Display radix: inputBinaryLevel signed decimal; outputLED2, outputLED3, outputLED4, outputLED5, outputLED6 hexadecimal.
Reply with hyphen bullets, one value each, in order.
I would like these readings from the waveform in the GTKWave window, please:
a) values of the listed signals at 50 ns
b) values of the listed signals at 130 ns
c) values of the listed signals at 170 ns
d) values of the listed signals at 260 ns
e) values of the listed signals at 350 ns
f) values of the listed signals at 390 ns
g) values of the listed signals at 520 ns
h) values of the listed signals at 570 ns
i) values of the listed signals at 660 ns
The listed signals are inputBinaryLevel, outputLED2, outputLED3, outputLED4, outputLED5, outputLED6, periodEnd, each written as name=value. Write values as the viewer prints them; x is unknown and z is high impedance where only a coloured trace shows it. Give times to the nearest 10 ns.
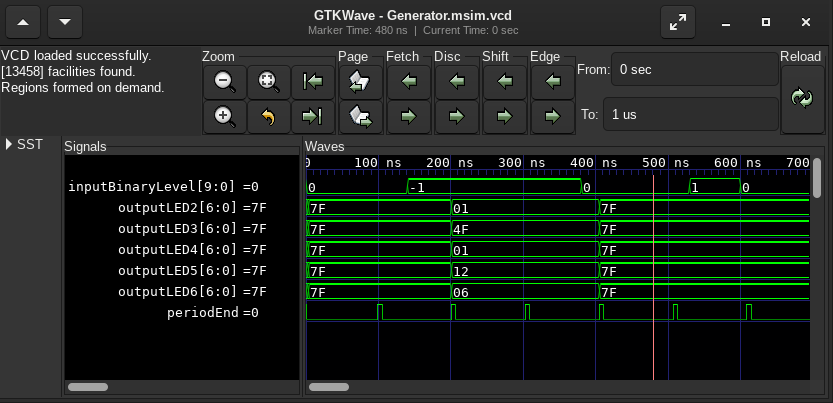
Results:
- inputBinaryLevel=0, outputLED2=7F, outputLED3=7F, outputLED4=7F, outputLED5=7F, outputLED6=7F, periodEnd=0
- inputBinaryLevel=0, outputLED2=7F, outputLED3=7F, outputLED4=7F, outputLED5=7F, outputLED6=7F, periodEnd=0
- inputBinaryLevel=-1, outputLED2=7F, outputLED3=7F, outputLED4=7F, outputLED5=7F, outputLED6=7F, periodEnd=0
- inputBinaryLevel=-1, outputLED2=01, outputLED3=4F, outputLED4=01, outputLED5=12, outputLED6=06, periodEnd=0
- inputBinaryLevel=-1, outputLED2=01, outputLED3=4F, outputLED4=01, outputLED5=12, outputLED6=06, periodEnd=0
- inputBinaryLevel=0, outputLED2=01, outputLED3=4F, outputLED4=01, outputLED5=12, outputLED6=06, periodEnd=0
- inputBinaryLevel=0, outputLED2=7F, outputLED3=7F, outputLED4=7F, outputLED5=7F, outputLED6=7F, periodEnd=0
- inputBinaryLevel=1, outputLED2=7F, outputLED3=7F, outputLED4=7F, outputLED5=7F, outputLED6=7F, periodEnd=0
- inputBinaryLevel=0, outputLED2=7F, outputLED3=7F, outputLED4=7F, outputLED5=7F, outputLED6=7F, periodEnd=0
